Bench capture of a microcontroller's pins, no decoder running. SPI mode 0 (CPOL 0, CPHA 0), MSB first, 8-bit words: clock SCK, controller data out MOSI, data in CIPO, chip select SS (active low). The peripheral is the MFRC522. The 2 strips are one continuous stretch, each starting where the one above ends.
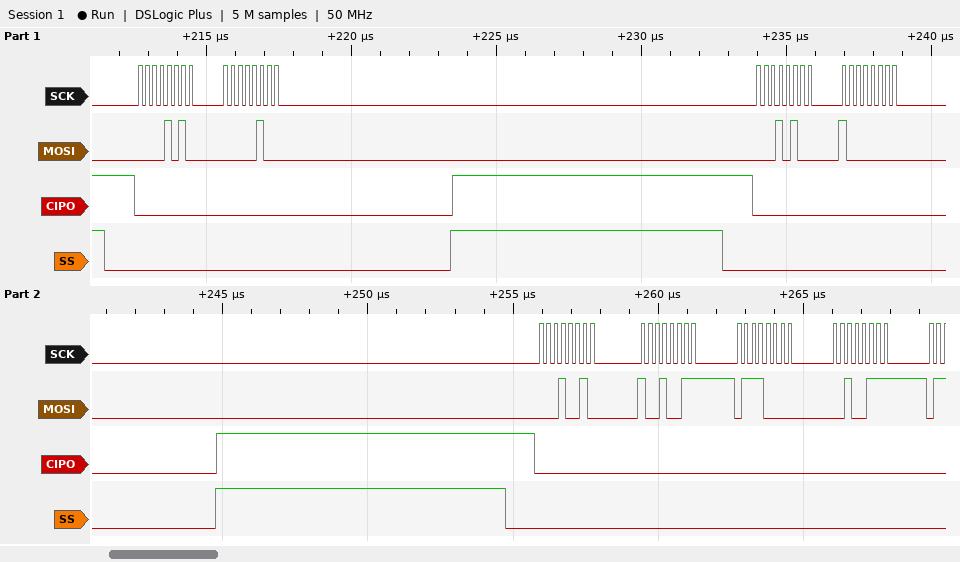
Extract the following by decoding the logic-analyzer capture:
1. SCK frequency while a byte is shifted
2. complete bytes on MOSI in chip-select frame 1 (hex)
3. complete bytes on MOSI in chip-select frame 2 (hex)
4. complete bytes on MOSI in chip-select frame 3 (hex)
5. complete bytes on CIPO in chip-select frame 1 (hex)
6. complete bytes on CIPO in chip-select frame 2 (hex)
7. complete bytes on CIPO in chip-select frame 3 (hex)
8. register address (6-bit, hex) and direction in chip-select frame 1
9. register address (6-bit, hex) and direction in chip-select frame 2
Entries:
4 MHz
0A 04
14 80
12 93 70 27
00 00
00 00
00 00 00 00
0x05 write
0x0A write
